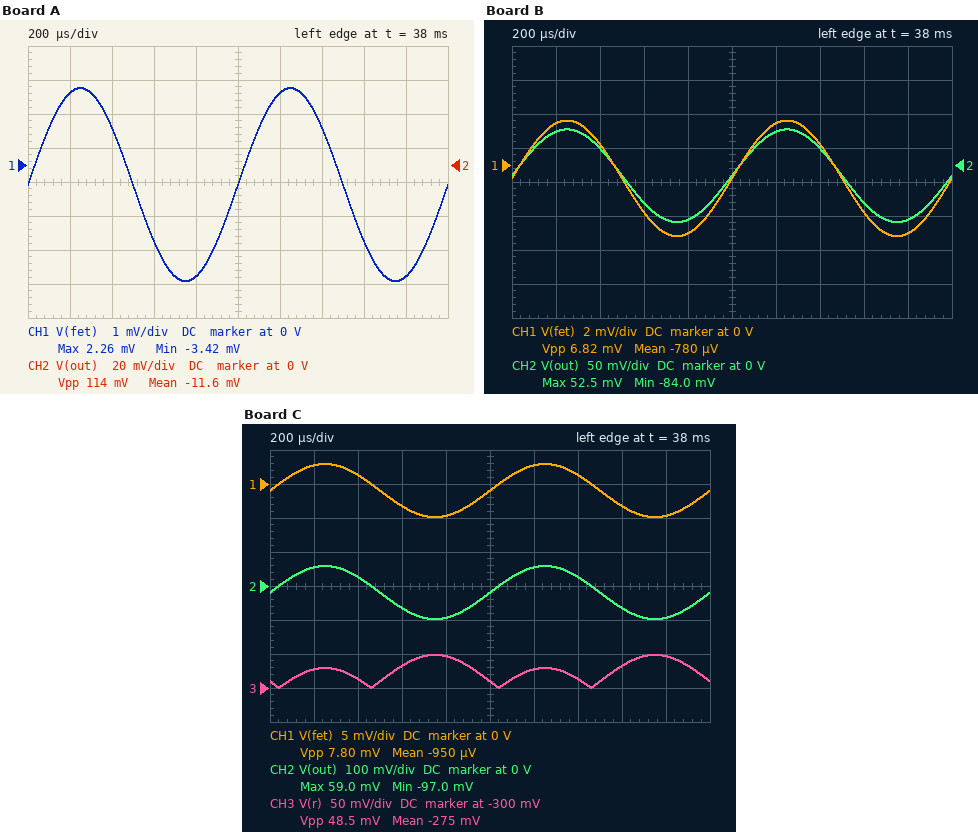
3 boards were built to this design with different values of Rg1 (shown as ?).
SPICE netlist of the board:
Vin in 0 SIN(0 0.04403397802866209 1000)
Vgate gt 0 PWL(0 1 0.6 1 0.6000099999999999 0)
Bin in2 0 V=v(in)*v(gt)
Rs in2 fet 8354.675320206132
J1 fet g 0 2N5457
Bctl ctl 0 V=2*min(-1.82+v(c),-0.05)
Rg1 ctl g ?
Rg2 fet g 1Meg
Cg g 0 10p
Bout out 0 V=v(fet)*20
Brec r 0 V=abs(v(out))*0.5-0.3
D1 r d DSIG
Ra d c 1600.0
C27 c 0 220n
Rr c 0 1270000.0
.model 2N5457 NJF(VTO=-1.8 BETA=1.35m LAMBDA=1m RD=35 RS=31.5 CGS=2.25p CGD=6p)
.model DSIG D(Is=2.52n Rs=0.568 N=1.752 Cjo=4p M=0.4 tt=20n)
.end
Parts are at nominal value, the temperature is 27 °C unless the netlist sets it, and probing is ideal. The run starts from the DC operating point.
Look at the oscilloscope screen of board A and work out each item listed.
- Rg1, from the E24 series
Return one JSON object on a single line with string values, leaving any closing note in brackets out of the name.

{"Rg1, from the E24 series": "2.4 MΩ"}
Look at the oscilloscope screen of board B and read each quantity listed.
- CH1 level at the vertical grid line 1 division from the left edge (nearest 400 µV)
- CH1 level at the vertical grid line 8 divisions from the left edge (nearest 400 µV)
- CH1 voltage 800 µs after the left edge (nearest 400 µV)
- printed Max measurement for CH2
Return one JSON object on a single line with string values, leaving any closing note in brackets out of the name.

{"CH1 level at the vertical grid line 1 division from the left edge": "2.4 mV", "CH1 level at the vertical grid line 8 divisions from the left edge": "-2.8 mV", "CH1 voltage 800 µs after the left edge": "-4.0 mV", "printed Max measurement for CH2": "52.5 mV"}
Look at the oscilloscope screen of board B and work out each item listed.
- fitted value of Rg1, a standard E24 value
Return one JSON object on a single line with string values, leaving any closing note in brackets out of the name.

{"fitted value of Rg1, a standard E24 value": "2 MΩ"}
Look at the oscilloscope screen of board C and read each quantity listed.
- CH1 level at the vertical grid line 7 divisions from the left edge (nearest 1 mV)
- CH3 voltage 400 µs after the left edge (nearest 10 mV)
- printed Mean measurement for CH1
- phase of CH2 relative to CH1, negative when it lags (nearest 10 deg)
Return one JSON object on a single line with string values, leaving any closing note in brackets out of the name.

{"CH1 level at the vertical grid line 7 divisions from the left edge": "1 mV", "CH3 voltage 400 µs after the left edge": "-290 mV", "printed Mean measurement for CH1": "-950 µV", "phase of CH2 relative to CH1, negative when it lags": "0 deg"}
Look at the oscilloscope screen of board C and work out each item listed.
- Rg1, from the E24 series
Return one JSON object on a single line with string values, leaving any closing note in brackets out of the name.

{"Rg1, from the E24 series": "1.8 MΩ"}
